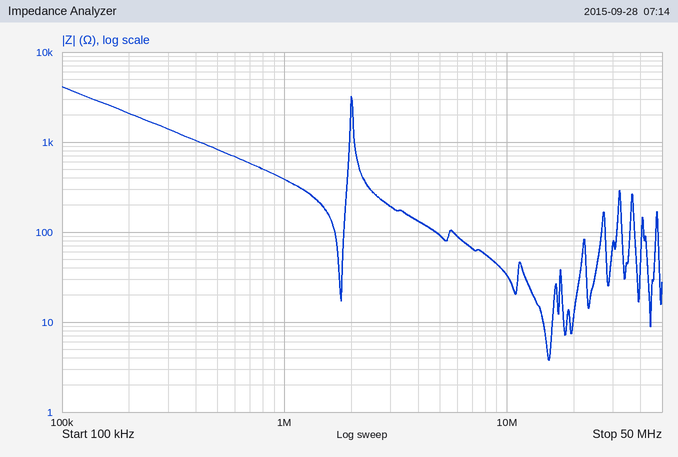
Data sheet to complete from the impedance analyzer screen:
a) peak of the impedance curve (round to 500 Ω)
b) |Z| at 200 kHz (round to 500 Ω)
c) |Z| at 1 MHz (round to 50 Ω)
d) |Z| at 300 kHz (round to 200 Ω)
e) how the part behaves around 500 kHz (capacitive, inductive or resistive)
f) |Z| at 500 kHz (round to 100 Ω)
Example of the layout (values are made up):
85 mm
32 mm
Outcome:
4.0 kΩ
2.0 kΩ
400 Ω
1.4 kΩ
capacitive
800 Ω
